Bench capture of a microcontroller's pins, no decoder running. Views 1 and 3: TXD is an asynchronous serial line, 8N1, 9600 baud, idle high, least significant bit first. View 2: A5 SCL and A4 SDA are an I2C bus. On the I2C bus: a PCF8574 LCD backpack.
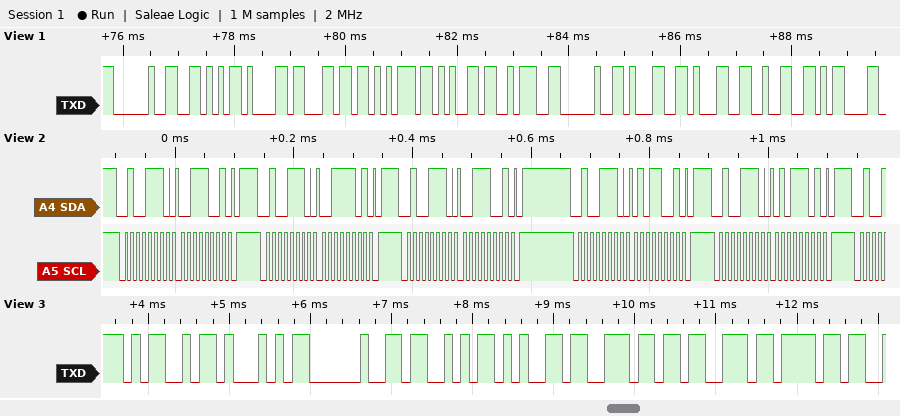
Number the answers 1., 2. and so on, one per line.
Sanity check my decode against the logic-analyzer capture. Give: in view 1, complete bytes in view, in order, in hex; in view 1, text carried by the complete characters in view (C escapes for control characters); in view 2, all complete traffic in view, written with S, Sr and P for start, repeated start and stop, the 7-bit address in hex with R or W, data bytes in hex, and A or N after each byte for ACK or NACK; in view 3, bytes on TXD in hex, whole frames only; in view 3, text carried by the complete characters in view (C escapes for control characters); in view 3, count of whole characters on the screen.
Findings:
1. 20 56 61 6C 75 65 3A 20 31 31 32 0D
2. " Value: 112\r"
3. S 27W A 39 A P S 27W A 3D A P S 27W A 39 A P S 27W A 59 A P S 27W A 5D A P
4. 4D 51 20 53 65 6E 73 6F
5. "MQ Senso"
6. 8
